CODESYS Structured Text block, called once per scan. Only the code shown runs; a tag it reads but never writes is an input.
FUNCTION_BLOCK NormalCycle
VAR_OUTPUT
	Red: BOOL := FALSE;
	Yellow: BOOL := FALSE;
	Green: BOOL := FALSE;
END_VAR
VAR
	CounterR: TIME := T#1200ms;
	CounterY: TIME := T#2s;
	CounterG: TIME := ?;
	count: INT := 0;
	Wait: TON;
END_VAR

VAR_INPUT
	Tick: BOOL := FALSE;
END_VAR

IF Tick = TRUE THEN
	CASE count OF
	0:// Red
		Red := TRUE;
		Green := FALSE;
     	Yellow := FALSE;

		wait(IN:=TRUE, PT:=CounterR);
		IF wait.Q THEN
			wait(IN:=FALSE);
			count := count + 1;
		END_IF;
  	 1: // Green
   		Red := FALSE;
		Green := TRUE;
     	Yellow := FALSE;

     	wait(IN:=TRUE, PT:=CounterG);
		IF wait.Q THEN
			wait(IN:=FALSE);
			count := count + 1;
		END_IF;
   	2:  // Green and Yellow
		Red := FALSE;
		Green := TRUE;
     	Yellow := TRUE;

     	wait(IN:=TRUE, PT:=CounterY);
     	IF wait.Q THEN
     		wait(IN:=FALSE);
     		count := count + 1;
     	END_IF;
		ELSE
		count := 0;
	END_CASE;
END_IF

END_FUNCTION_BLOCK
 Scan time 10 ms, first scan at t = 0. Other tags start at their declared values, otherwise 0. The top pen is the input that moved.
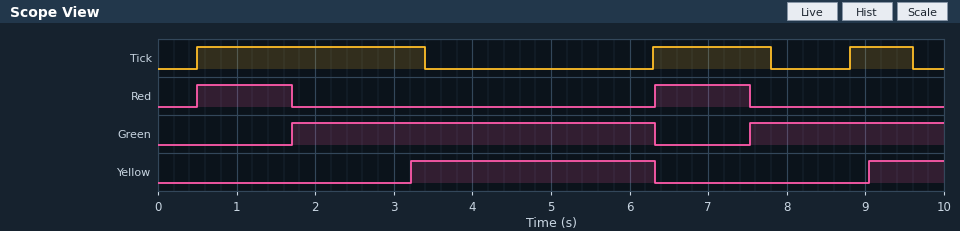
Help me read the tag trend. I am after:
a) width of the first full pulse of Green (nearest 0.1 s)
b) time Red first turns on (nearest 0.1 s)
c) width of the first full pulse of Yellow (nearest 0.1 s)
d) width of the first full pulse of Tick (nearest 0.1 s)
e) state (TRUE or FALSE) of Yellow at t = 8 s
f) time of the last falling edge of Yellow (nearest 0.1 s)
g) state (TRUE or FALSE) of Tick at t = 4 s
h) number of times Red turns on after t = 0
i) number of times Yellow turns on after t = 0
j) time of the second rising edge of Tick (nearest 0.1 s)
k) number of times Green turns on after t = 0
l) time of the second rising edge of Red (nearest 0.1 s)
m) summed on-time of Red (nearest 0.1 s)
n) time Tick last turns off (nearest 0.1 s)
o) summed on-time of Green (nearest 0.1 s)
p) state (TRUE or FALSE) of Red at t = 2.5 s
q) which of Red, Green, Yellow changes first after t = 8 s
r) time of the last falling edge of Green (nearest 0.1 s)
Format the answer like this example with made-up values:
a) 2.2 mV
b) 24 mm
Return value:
a) 4.6 s
b) 0.5 s
c) 3.1 s
d) 2.9 s
e) FALSE
f) 6.3 s
g) FALSE
h) 2
i) 2
j) 6.3 s
k) 2
l) 6.3 s
m) 2.4 s
n) 9.6 s
o) 7.1 s
p) FALSE
q) Yellow
r) 6.3 s
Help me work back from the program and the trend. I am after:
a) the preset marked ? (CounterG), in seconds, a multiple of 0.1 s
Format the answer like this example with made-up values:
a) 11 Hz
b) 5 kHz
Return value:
a) 1.5 s
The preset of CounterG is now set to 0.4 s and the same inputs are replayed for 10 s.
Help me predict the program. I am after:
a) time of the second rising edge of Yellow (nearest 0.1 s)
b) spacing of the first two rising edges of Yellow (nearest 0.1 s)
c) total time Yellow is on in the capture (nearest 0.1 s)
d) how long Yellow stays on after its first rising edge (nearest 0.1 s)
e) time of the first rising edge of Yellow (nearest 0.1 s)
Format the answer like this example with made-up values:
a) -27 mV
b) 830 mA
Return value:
a) 8.8 s
b) 6.7 s
c) 5.4 s
d) 4.2 s
e) 2.1 s
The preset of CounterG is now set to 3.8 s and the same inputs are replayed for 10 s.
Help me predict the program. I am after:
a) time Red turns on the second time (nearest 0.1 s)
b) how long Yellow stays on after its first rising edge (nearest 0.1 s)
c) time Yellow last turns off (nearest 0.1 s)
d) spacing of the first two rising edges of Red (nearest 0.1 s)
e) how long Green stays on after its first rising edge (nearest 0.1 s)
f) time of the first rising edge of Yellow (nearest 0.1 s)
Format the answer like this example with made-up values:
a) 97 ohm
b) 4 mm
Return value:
a) 8.8 s
b) 2.5 s
c) 8.8 s
d) 8.3 s
e) 7.1 s
f) 6.3 s
